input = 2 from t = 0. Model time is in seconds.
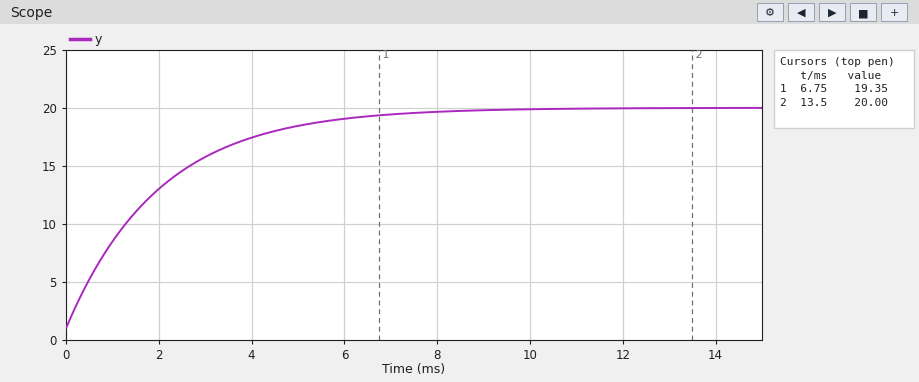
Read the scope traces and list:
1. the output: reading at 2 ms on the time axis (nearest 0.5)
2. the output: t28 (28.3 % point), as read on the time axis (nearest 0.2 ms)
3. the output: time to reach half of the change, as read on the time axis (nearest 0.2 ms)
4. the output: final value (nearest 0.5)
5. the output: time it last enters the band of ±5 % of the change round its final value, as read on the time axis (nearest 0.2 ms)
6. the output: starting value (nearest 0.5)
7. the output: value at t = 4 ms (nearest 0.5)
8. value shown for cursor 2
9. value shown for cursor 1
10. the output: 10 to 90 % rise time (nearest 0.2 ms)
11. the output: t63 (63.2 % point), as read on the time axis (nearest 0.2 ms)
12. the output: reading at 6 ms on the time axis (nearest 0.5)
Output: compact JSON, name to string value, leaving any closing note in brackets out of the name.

{"the output: reading at 2 ms on the time axis": "13.0", "the output: t28 (28.3 % point), as read on the time axis": "0.6 ms", "the output: time to reach half of the change, as read on the time axis": "1.4 ms", "the output: final value": "20.0", "the output: time it last enters the band of ±5 % of the change round its final value, as read on the time axis": "6.0 ms", "the output: starting value": "1.0", "the output: value at t = 4 ms": "17.5", "value shown for cursor 2": "20.00", "value shown for cursor 1": "19.35", "the output: 10 to 90 % rise time": "4.4 ms", "the output: t63 (63.2 % point), as read on the time axis": "2.0 ms", "the output: reading at 6 ms on the time axis": "19.0"}
